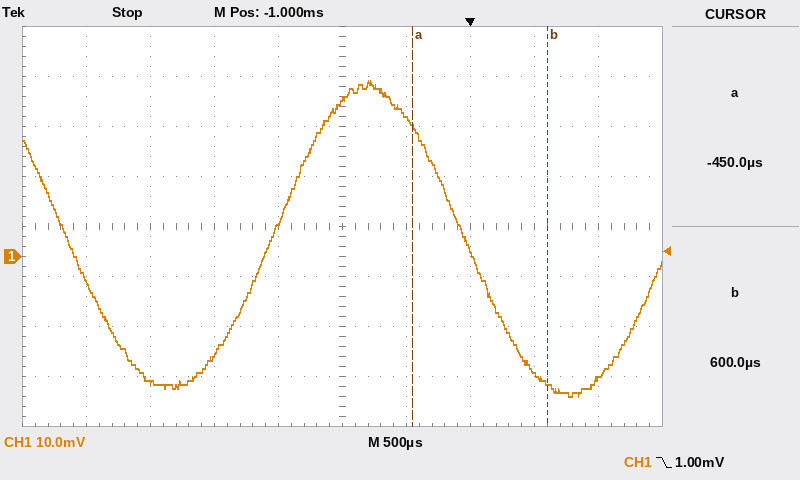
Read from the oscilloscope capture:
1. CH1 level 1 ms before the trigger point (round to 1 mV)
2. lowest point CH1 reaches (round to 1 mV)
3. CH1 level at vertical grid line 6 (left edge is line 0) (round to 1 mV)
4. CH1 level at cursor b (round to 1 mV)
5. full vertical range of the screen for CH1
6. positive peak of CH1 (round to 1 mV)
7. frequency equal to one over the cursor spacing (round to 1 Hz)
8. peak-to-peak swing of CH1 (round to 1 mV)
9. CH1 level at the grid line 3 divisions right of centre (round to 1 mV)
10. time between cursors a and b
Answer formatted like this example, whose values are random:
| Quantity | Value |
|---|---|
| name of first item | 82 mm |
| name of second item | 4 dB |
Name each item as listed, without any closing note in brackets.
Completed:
| Quantity | Value |
|---|---|
| CH1 level 1 ms before the trigger point | 31 mV |
| lowest point CH1 reaches | -28 mV |
| CH1 level at vertical grid line 6 (left edge is line 0) | 28 mV |
| CH1 level at cursor b | -25 mV |
| full vertical range of the screen for CH1 | 80 mV |
| positive peak of CH1 | 35 mV |
| frequency equal to one over the cursor spacing | 952 Hz |
| peak-to-peak swing of CH1 | 63 mV |
| CH1 level at the grid line 3 divisions right of centre | -23 mV |
| time between cursors a and b | 1.05 ms |
